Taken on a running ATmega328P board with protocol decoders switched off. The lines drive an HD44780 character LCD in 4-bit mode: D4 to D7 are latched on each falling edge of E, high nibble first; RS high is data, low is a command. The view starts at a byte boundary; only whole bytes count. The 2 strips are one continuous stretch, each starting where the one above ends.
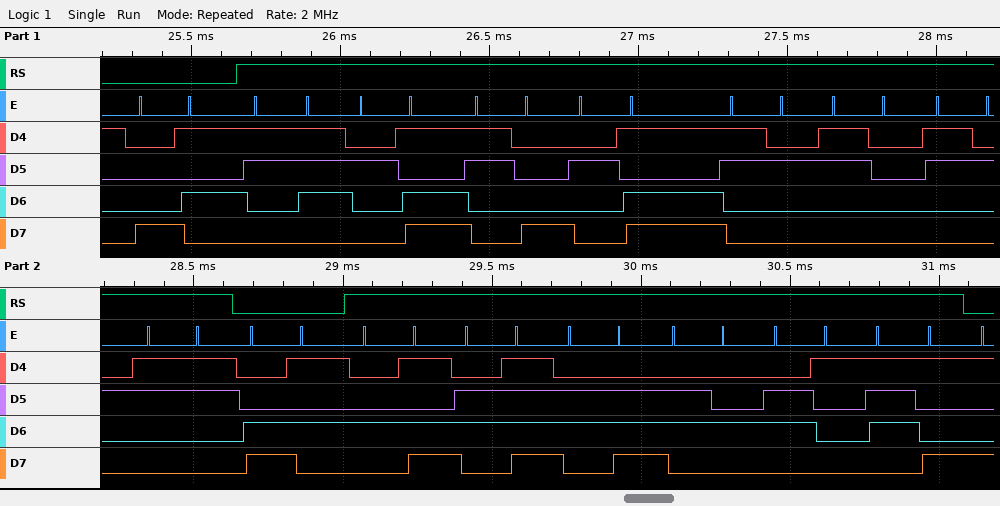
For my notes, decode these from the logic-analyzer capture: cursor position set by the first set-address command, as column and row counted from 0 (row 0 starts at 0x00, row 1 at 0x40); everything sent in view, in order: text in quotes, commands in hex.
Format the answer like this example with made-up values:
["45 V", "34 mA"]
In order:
["column 5, row 0", "0x85 \"7-8-2023\" 0xC5 \"Monday\""]
